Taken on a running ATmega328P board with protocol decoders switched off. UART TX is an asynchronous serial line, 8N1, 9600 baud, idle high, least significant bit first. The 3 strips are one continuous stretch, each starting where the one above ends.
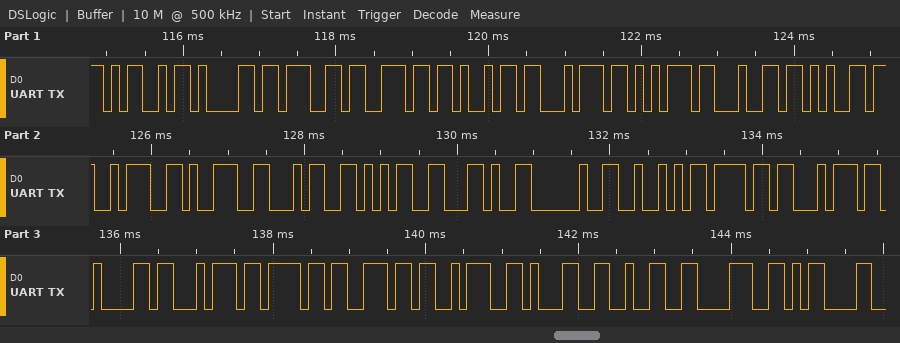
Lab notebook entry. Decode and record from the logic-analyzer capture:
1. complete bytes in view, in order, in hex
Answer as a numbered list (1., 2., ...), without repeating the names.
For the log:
1. 4D 61 67 6E 69 74 75 64 65 3A 39 34 35 2C 20 52 6F 74 61 74 6F 6E 3A 31 32 38 0D
